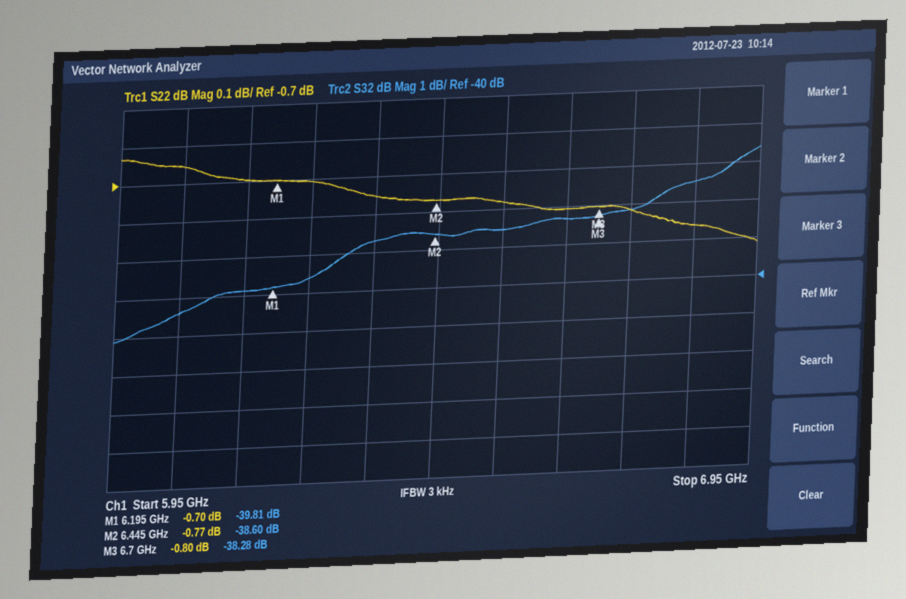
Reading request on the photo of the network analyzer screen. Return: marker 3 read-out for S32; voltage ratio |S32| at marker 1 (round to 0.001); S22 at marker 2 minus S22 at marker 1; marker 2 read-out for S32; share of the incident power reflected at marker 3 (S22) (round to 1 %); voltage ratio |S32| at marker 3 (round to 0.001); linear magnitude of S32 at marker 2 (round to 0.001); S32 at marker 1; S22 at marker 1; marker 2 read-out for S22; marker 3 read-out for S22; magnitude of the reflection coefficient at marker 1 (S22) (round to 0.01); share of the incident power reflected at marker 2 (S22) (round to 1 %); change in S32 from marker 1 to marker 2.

-38.28 dB
0.010
-0.07 dB
-38.60 dB
83 %
0.012
0.012
-39.81 dB
-0.70 dB
-0.77 dB
-0.80 dB
0.92
84 %
1.21 dB
